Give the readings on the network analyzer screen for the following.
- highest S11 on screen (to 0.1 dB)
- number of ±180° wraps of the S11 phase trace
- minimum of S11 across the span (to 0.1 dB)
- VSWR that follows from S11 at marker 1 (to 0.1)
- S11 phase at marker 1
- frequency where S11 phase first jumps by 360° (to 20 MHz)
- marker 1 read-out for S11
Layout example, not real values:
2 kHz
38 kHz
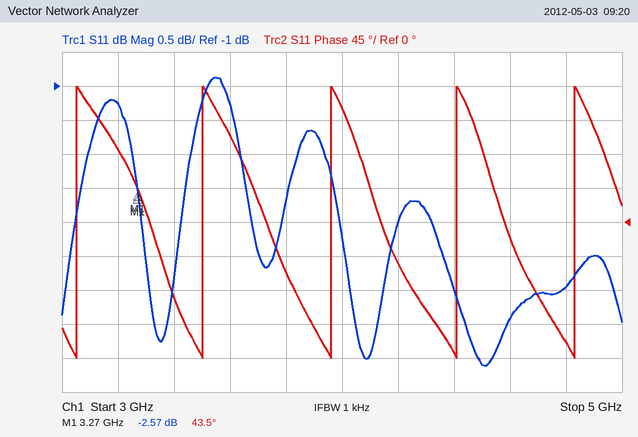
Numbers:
-0.9 dB
5
-5.1 dB
6.8
43.5°
3.06 GHz
-2.57 dB
